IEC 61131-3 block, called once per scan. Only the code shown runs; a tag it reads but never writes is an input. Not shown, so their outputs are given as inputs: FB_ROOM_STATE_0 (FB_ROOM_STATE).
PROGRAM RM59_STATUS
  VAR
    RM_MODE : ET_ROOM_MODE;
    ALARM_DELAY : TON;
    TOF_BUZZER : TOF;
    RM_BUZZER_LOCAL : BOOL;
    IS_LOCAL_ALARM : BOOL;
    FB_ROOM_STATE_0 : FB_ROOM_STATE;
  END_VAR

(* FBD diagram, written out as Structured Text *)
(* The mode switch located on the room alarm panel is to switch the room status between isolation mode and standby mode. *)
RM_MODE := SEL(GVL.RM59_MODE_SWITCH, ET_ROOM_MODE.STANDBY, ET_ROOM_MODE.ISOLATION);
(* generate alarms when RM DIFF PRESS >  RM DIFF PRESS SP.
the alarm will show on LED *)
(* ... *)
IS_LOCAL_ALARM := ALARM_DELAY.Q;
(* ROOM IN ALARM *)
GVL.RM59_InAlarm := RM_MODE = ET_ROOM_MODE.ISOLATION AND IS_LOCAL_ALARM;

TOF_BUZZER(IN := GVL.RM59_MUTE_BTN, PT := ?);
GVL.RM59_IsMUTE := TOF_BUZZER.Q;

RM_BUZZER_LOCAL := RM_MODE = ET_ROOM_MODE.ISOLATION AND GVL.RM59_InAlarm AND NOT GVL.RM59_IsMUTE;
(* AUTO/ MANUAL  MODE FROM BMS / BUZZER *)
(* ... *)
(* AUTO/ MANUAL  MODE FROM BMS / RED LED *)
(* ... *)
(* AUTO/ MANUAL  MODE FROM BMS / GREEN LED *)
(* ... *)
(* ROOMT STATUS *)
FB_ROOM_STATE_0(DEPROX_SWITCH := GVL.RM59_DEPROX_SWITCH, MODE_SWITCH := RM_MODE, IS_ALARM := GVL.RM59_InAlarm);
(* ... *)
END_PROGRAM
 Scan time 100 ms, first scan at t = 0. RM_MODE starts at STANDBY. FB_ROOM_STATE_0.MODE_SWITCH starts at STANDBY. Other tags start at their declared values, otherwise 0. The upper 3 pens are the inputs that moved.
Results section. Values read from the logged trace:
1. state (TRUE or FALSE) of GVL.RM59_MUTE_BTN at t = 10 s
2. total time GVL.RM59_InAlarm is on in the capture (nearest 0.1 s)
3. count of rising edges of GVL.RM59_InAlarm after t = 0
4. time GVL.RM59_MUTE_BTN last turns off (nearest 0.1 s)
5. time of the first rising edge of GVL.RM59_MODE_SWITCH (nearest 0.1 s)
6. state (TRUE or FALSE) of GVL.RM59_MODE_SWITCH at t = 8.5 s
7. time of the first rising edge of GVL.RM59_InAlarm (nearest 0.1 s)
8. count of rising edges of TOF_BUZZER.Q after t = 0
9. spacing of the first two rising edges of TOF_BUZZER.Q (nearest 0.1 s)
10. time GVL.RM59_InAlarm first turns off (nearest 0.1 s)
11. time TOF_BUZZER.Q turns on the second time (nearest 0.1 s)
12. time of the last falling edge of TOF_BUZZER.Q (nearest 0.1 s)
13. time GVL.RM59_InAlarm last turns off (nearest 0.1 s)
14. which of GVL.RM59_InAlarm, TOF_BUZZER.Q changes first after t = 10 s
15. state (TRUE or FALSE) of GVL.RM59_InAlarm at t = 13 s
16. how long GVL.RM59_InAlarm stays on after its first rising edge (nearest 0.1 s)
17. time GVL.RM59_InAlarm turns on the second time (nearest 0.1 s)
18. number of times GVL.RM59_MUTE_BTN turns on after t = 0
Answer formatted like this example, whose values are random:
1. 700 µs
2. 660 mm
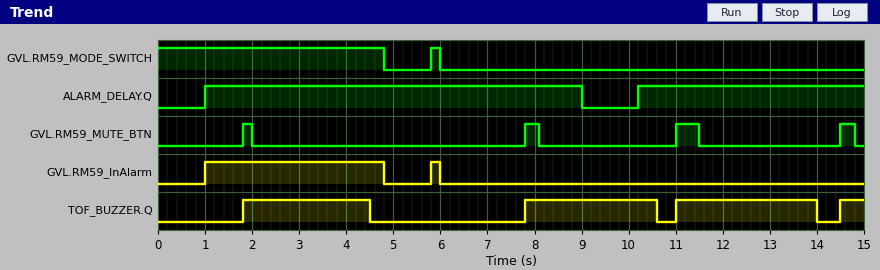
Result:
1. FALSE
2. 4.0 s
3. 2
4. 14.8 s
5. 5.8 s
6. FALSE
7. 1.0 s
8. 4
9. 6.0 s
10. 4.8 s
11. 7.8 s
12. 14.0 s
13. 6.0 s
14. TOF_BUZZER.Q
15. FALSE
16. 3.8 s
17. 5.8 s
18. 4
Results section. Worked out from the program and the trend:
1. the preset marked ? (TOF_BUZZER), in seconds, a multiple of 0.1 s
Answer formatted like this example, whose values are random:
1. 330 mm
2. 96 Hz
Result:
1. 2.5 s
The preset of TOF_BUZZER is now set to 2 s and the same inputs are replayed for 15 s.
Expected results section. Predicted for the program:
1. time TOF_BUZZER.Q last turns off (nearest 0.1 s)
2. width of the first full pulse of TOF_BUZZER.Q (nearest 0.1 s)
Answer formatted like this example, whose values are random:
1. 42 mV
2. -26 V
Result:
1. 13.5 s
2. 2.2 s
